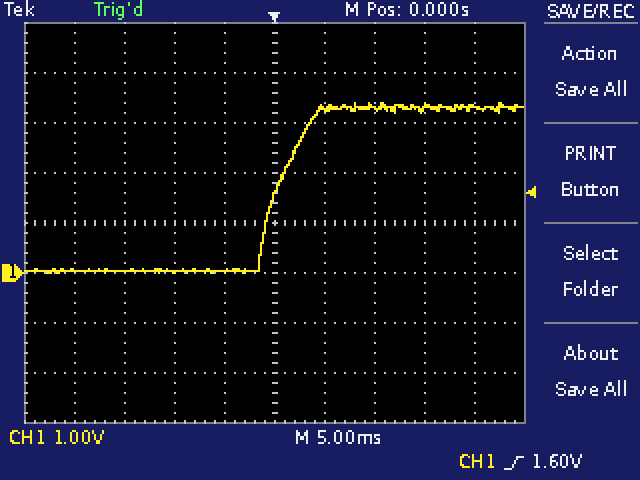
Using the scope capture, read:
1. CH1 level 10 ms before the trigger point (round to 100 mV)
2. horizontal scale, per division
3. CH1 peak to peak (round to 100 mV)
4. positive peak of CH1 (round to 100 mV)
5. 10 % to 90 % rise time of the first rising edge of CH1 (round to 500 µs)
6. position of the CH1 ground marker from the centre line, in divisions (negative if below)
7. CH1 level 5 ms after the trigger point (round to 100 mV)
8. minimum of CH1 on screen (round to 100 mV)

0.0 V
5 ms
3.4 V
3.4 V
5.0 ms
-1.0 div
3.3 V
0.0 V
